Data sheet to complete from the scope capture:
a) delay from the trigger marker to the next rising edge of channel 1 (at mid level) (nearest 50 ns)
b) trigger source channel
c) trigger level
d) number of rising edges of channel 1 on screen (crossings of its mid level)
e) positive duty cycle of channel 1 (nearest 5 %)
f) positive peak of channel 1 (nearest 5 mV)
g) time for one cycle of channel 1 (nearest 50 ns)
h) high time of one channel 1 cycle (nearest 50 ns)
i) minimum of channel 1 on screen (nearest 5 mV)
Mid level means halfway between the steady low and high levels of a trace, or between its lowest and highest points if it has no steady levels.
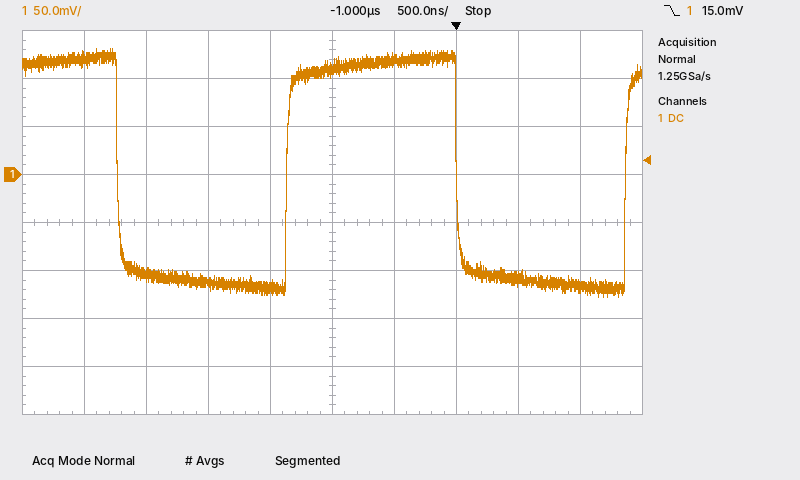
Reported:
1.35 µs
channel 1
15.0 mV
2
50 %
130 mV
2.75 µs
1.35 µs
-125 mV
